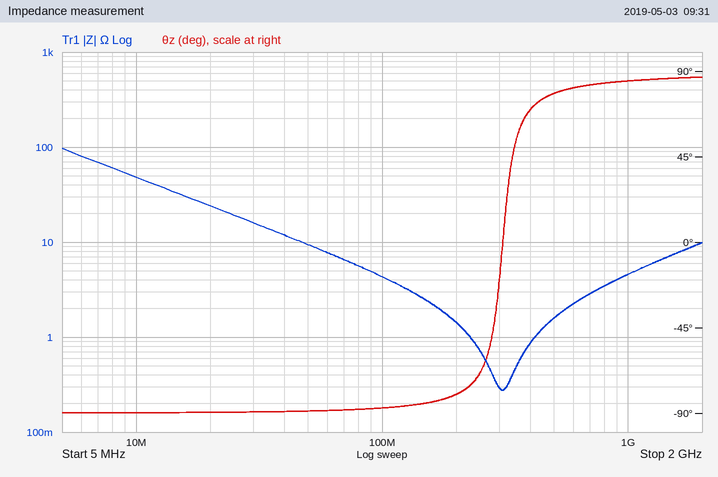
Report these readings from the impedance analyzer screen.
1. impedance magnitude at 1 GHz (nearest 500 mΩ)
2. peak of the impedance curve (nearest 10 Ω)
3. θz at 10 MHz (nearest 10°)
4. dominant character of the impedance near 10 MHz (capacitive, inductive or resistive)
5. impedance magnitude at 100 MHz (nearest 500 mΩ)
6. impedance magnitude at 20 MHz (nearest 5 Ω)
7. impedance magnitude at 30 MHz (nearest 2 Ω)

4.5 Ω
100 Ω
-90°
capacitive
4.5 Ω
25 Ω
16 Ω
